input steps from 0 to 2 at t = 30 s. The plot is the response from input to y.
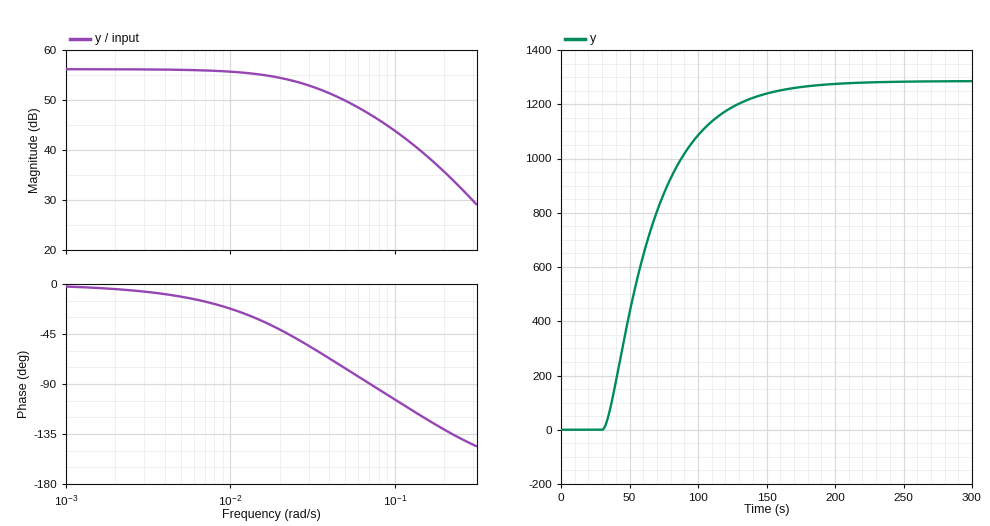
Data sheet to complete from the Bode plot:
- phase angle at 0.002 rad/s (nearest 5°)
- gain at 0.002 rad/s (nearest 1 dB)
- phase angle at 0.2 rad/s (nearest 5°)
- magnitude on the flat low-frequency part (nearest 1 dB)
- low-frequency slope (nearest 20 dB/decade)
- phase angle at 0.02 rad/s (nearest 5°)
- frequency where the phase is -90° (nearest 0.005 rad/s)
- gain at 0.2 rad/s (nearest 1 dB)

-5°
56 dB
-130°
56 dB
0 dB/decade
-40°
0.070 rad/s
36 dB
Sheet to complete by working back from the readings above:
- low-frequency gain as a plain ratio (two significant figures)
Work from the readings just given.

630
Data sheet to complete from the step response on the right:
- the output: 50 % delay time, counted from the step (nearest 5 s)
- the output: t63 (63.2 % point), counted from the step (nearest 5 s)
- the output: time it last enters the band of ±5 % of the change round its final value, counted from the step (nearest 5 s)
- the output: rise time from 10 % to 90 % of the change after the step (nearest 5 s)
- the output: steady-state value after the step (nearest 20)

30 s
40 s
110 s
75 s
1280
